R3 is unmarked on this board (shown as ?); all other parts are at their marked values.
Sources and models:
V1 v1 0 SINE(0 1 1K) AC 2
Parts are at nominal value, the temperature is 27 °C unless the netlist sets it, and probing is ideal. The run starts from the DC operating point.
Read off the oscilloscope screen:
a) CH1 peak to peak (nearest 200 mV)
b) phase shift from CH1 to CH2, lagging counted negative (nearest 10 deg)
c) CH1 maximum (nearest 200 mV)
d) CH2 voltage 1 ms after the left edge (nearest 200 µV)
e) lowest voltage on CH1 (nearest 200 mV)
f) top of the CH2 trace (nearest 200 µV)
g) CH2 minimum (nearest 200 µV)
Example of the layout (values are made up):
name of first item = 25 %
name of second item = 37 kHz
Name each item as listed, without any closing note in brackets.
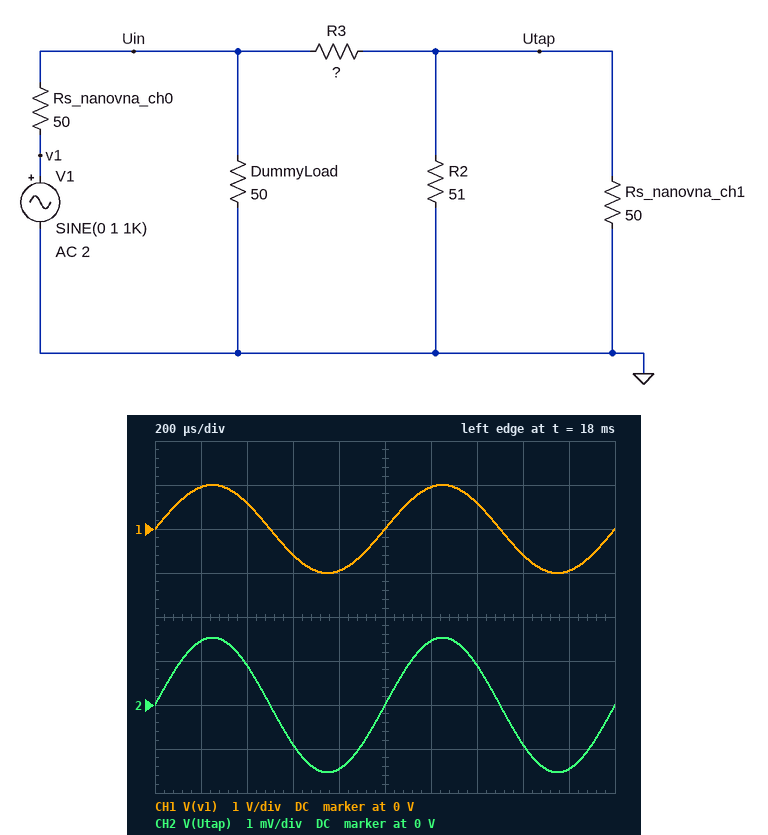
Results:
CH1 peak to peak = 2.0 V
phase shift from CH1 to CH2, lagging counted negative = 0 deg
CH1 maximum = 1.0 V
CH2 voltage 1 ms after the left edge = 0 V
lowest voltage on CH1 = -1.0 V
top of the CH2 trace = 1.6 mV
CH2 minimum = -1.6 mV
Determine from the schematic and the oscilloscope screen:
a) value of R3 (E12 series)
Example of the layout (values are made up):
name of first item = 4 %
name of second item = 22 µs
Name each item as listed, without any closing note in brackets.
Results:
value of R3 = 8.2 kΩ
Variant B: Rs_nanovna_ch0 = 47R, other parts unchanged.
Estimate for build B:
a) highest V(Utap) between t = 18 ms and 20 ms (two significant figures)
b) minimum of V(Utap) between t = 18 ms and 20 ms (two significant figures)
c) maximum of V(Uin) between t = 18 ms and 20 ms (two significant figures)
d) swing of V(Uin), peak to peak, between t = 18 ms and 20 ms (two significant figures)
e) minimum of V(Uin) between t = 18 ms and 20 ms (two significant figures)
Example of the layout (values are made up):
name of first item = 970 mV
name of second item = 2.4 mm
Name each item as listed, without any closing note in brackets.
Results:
highest V(Utap) between t = 18 ms and 20 ms = 1.6 mV
minimum of V(Utap) between t = 18 ms and 20 ms = -1.6 mV
maximum of V(Uin) between t = 18 ms and 20 ms = 510 mV
swing of V(Uin), peak to peak, between t = 18 ms and 20 ms = 1.0 V
minimum of V(Uin) between t = 18 ms and 20 ms = -510 mV
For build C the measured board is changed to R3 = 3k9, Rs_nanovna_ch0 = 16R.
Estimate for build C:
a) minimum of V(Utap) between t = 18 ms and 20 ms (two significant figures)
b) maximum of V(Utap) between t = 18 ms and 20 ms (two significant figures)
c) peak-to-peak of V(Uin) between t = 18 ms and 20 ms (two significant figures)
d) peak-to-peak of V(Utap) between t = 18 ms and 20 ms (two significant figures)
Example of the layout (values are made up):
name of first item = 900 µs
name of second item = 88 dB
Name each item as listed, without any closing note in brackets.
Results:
minimum of V(Utap) between t = 18 ms and 20 ms = -4.9 mV
maximum of V(Utap) between t = 18 ms and 20 ms = 4.9 mV
peak-to-peak of V(Uin) between t = 18 ms and 20 ms = 1.5 V
peak-to-peak of V(Utap) between t = 18 ms and 20 ms = 9.7 mV
